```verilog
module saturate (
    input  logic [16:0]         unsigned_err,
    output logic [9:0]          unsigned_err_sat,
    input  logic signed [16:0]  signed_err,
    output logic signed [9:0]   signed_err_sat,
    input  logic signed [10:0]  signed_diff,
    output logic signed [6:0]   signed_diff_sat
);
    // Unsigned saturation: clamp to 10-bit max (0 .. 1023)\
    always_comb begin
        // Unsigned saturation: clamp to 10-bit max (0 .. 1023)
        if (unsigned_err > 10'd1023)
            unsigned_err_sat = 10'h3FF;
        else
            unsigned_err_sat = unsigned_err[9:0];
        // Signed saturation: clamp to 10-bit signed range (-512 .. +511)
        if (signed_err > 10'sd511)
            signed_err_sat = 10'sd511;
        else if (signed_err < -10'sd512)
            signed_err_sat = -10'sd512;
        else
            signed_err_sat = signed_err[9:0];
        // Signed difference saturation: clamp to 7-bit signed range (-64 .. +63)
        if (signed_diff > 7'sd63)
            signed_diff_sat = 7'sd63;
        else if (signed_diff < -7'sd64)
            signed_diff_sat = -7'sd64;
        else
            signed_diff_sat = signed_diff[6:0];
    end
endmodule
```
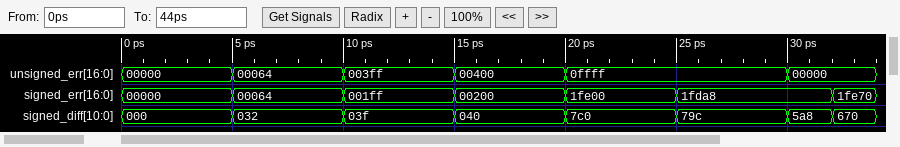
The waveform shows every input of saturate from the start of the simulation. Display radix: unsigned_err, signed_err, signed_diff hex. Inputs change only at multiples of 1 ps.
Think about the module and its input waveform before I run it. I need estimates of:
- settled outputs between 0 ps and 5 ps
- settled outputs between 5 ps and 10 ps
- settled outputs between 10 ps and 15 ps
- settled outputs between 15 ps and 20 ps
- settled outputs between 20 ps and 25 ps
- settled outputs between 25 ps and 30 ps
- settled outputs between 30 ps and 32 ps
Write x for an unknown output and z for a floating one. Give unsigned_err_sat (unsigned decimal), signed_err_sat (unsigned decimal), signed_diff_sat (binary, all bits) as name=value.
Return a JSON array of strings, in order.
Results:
["unsigned_err_sat=0, signed_err_sat=512, signed_diff_sat=1000000", "unsigned_err_sat=100, signed_err_sat=512, signed_diff_sat=1000000", "unsigned_err_sat=1023, signed_err_sat=512, signed_diff_sat=1000000", "unsigned_err_sat=1023, signed_err_sat=511, signed_diff_sat=0111111", "unsigned_err_sat=1023, signed_err_sat=512, signed_diff_sat=1000000", "unsigned_err_sat=1023, signed_err_sat=512, signed_diff_sat=1000000", "unsigned_err_sat=0, signed_err_sat=512, signed_diff_sat=1000000"]
